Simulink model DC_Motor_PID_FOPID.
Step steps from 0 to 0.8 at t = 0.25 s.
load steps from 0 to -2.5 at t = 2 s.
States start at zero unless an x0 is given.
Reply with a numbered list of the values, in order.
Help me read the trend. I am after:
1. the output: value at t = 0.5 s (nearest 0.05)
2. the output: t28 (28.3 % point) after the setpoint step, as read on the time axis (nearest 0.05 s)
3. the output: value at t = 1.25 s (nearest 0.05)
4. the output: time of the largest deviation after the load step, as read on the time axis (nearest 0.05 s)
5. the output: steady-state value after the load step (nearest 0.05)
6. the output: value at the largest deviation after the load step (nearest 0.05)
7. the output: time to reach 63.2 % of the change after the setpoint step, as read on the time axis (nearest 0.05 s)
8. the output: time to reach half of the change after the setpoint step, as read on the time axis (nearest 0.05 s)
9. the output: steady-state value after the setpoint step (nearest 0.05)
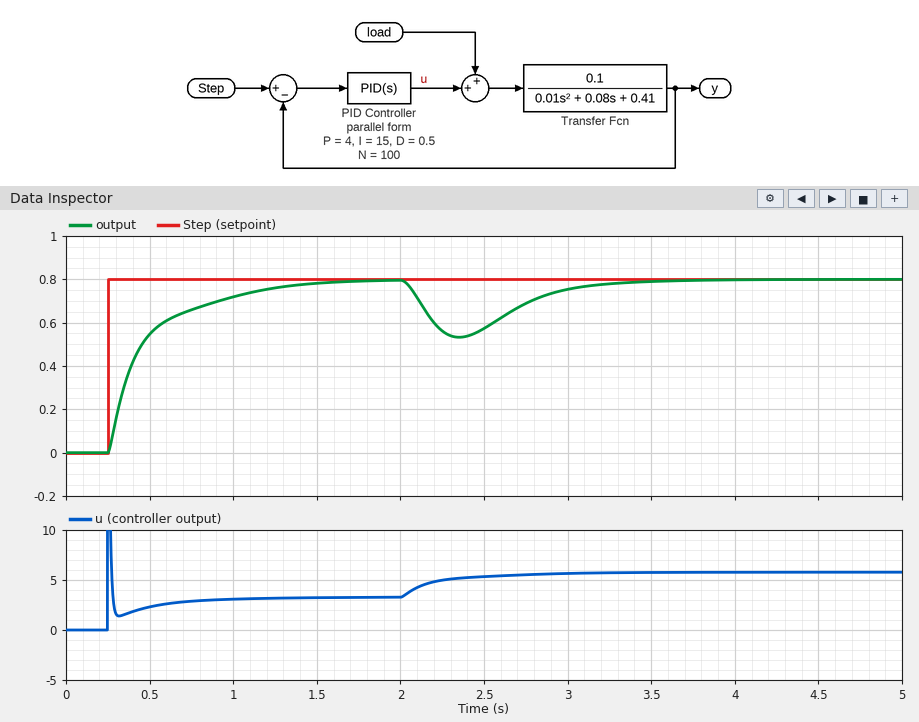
1. 0.55
2. 0.30 s
3. 0.75
4. 2.35 s
5. 0.80
6. 0.55
7. 0.45 s
8. 0.40 s
9. 0.80
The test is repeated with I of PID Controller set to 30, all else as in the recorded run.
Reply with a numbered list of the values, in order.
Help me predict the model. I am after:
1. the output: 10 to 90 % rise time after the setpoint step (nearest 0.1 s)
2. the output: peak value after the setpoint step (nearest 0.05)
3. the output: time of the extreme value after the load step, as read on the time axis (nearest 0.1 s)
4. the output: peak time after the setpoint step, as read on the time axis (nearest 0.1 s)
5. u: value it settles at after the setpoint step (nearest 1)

1. 0.3 s
2. 0.85
3. 2.3 s
4. 0.8 s
5. 3
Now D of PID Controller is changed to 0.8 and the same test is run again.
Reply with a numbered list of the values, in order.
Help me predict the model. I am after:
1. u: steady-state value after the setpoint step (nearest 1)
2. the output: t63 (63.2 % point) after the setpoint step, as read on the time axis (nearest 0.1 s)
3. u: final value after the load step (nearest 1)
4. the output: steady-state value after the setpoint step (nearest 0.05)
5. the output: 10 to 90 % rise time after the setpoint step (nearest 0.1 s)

1. 3
2. 0.4 s
3. 6
4. 0.80
5. 0.8 s
